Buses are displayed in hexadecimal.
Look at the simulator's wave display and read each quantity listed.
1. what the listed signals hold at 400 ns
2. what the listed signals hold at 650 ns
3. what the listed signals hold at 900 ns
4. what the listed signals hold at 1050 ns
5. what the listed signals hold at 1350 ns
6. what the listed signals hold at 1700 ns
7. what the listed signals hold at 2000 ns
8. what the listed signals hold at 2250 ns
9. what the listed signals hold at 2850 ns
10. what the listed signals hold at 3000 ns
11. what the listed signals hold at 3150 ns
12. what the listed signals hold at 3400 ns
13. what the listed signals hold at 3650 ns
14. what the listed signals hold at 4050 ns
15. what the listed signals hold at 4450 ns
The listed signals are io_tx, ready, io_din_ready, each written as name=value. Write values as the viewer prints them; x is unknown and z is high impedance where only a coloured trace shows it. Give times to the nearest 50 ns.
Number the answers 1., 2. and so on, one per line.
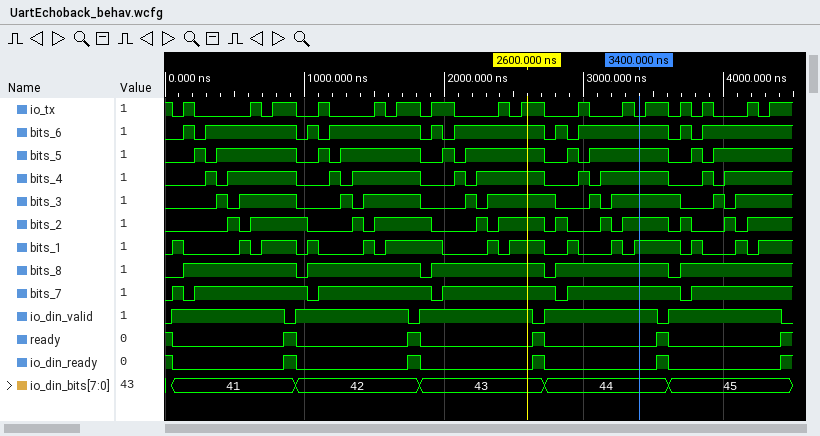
1. io_tx=0, ready=0, io_din_ready=0
2. io_tx=1, ready=0, io_din_ready=0
3. io_tx=1, ready=1, io_din_ready=1
4. io_tx=0, ready=0, io_din_ready=0
5. io_tx=0, ready=0, io_din_ready=0
6. io_tx=1, ready=0, io_din_ready=0
7. io_tx=1, ready=0, io_din_ready=0
8. io_tx=0, ready=0, io_din_ready=0
9. io_tx=0, ready=0, io_din_ready=0
10. io_tx=1, ready=0, io_din_ready=0
11. io_tx=0, ready=0, io_din_ready=0
12. io_tx=0, ready=0, io_din_ready=0
13. io_tx=0, ready=0, io_din_ready=0
14. io_tx=0, ready=0, io_din_ready=0
15. io_tx=1, ready=1, io_din_ready=1
